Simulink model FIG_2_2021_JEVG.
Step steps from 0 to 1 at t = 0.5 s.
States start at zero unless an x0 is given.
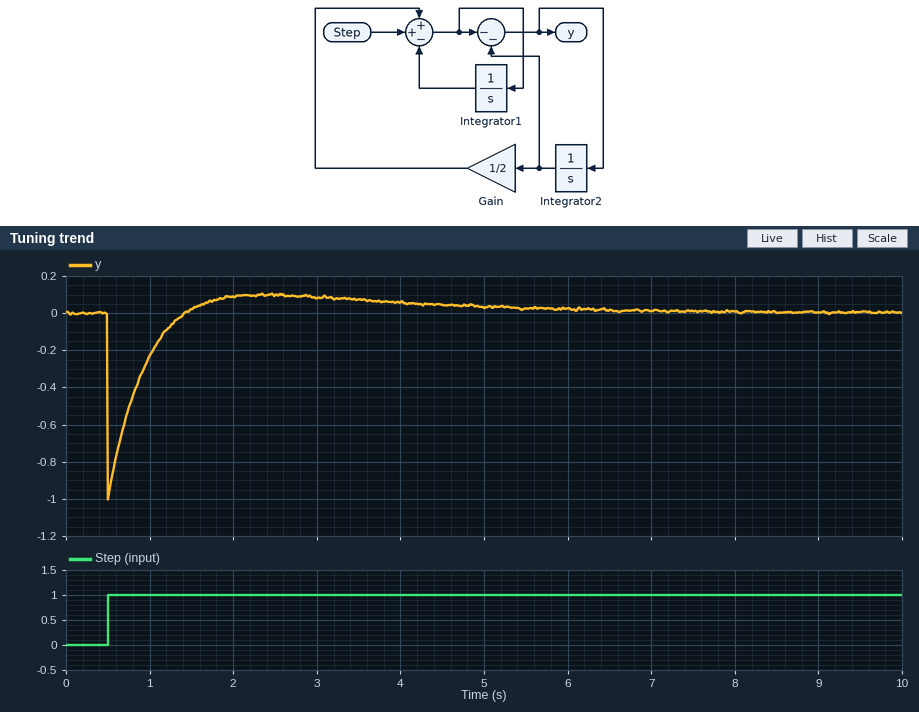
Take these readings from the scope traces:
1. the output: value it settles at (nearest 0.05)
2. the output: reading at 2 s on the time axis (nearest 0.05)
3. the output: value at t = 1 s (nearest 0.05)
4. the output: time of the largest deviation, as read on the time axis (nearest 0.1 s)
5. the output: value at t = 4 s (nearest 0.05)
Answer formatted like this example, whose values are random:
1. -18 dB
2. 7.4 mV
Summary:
1. 0.00
2. 0.10
3. -0.25
4. 0.5 s
5. 0.05
